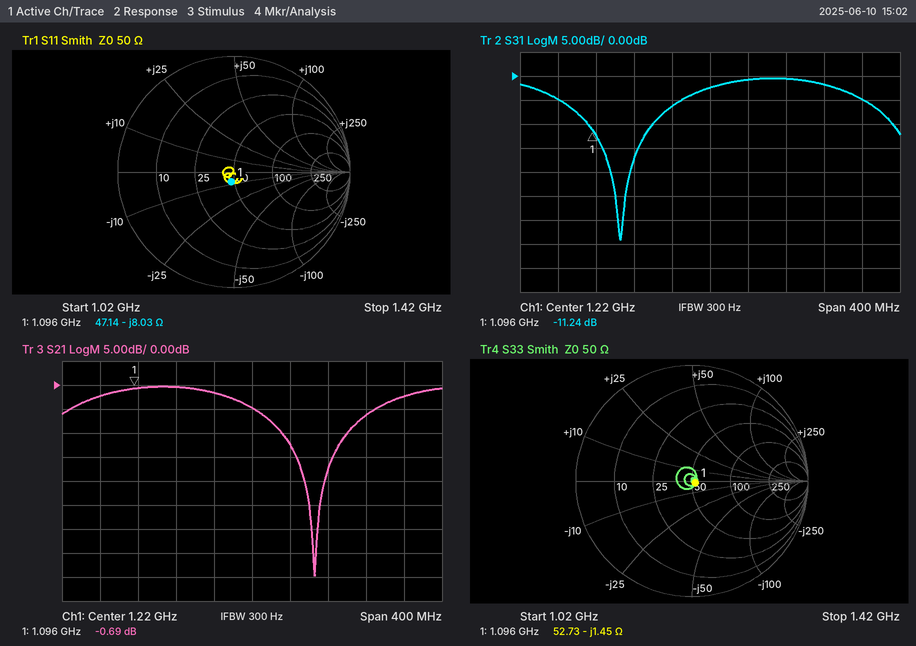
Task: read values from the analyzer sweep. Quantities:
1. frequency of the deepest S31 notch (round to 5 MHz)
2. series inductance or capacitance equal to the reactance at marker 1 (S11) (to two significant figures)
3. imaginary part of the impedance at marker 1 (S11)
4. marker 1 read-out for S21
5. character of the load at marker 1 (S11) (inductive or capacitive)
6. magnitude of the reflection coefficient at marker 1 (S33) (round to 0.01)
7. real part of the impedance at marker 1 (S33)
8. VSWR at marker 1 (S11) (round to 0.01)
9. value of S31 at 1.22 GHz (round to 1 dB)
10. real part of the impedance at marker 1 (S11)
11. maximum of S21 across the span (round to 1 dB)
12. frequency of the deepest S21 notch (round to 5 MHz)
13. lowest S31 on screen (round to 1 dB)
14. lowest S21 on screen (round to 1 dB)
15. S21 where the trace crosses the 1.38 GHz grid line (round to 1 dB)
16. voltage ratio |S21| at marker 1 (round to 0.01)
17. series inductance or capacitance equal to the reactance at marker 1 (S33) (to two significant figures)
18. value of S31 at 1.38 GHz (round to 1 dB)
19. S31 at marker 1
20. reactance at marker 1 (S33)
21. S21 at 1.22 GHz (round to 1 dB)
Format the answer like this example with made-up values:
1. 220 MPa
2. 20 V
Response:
1. 1.125 GHz
2. 18 pF
3. -8.03 Ω
4. -0.69 dB
5. capacitive
6. 0.03
7. 52.73 Ω
8. 1.19
9. -2 dB
10. 47.14 Ω
11. 0 dB
12. 1.285 GHz
13. -34 dB
14. -40 dB
15. -2 dB
16. 0.92
17. 100 pF
18. -5 dB
19. -11.24 dB
20. -1.45 Ω
21. -5 dB
